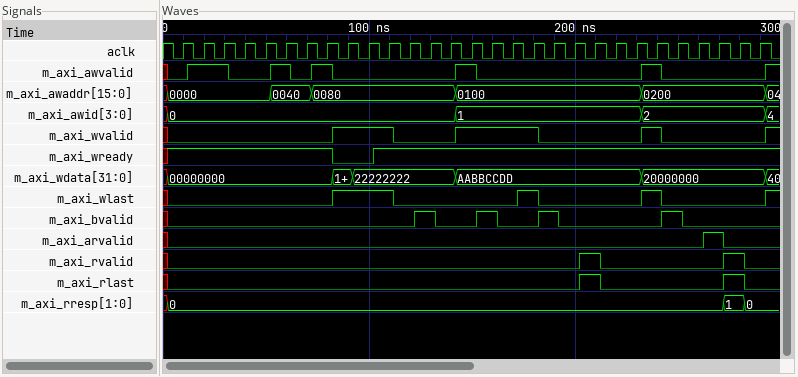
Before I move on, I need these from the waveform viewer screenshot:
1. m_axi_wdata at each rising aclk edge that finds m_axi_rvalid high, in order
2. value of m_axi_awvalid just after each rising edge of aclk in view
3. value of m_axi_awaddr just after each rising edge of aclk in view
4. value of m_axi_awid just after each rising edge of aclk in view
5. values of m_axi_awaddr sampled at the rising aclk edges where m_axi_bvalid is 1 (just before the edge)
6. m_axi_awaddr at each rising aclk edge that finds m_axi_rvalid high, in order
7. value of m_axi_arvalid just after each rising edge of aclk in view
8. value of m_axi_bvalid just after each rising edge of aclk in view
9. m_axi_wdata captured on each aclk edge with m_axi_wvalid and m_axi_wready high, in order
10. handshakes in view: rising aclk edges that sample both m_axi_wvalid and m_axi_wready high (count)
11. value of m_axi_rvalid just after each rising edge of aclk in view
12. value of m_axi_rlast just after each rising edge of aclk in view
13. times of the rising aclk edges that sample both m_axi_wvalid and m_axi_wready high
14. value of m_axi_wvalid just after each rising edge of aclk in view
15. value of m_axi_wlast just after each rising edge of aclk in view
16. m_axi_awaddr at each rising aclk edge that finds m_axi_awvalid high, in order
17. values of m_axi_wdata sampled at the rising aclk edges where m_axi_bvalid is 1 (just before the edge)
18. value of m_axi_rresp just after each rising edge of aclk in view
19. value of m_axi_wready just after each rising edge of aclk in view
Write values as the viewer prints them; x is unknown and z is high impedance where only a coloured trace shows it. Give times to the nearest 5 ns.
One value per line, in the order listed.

AABBCCDD, 20000000
0 1 1 0 0 1 0 1 0 0 0 0 0 0 1 0 0 0 0 0 0 0 0 1 0 0 0 0 0
0000, 0000, 0000, 0000, 0000, 0040, 0040, 0080, 0080, 0080, 0080, 0080, 0080, 0080, 0100, 0100, 0100, 0100, 0100, 0100, 0100, 0100, 0100, 0200, 0200, 0200, 0200, 0200, 0200
0, 0, 0, 0, 0, 0, 0, 0, 0, 0, 0, 0, 0, 0, 1, 1, 1, 1, 1, 1, 1, 1, 1, 2, 2, 2, 2, 2, 2
0080, 0100, 0100, 0200
0100, 0200
0 0 0 0 0 0 0 0 0 0 0 0 0 0 0 0 0 0 0 0 0 0 0 0 0 0 1 0 0
0 0 0 0 0 0 0 0 0 0 0 0 1 0 0 1 0 0 1 0 0 0 0 0 1 0 0 0 0
22222222, AABBCCDD, AABBCCDD, AABBCCDD, AABBCCDD, 20000000
6
0 0 0 0 0 0 0 0 0 0 0 0 0 0 0 0 0 0 0 0 1 0 0 0 0 0 0 1 0
0 0 0 0 0 0 0 0 0 0 0 0 0 0 0 0 0 0 0 0 1 0 0 0 0 0 0 1 0
110 ns, 150 ns, 160 ns, 170 ns, 180 ns, 240 ns
0 0 0 0 0 0 0 0 1 1 1 0 0 0 1 1 1 1 0 0 0 0 0 1 0 0 0 0 0
0 0 0 0 0 0 0 0 1 1 1 0 0 0 0 0 0 1 0 0 0 0 0 1 0 0 0 0 0
0000, 0000, 0040, 0080, 0100, 0200
22222222, AABBCCDD, AABBCCDD, 20000000
0, 0, 0, 0, 0, 0, 0, 0, 0, 0, 0, 0, 0, 0, 0, 0, 0, 0, 0, 0, 0, 0, 0, 0, 0, 0, 0, 1, 0
1 1 1 1 1 1 1 1 0 0 1 1 1 1 1 1 1 1 1 1 1 1 1 1 1 1 1 1 1
